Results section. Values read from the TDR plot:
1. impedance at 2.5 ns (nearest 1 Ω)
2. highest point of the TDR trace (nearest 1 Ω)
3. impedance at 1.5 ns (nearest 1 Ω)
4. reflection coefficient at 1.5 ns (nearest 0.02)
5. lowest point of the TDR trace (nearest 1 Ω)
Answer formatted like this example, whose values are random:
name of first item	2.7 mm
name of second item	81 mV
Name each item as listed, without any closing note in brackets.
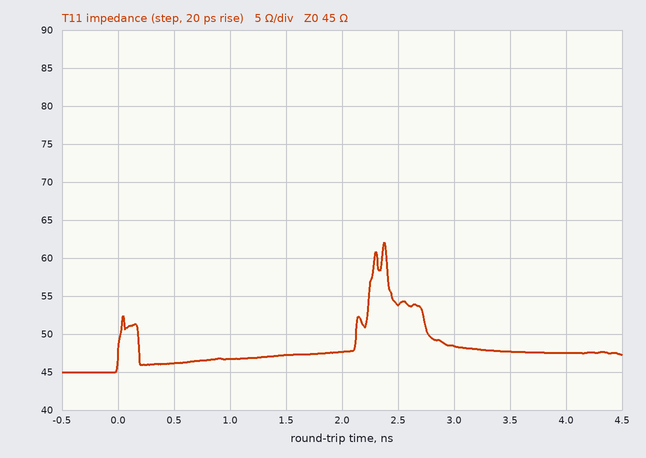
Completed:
impedance at 2.5 ns	54 Ω
highest point of the TDR trace	62 Ω
impedance at 1.5 ns	47 Ω
reflection coefficient at 1.5 ns	+0.02
lowest point of the TDR trace	45 Ω
